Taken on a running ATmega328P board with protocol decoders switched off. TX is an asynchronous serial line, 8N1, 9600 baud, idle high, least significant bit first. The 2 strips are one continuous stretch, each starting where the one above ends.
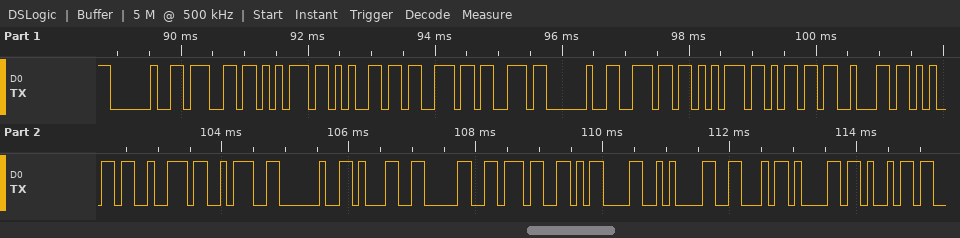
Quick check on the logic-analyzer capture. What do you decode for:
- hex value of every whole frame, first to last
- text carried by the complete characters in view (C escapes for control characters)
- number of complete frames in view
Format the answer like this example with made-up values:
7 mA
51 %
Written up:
20 67 75 65 73 73 20 6E 75 6D 62 65 72 3A 20 31 30 37 0D 0A 46 61 69
" guess number: 107\r\nFai"
23
